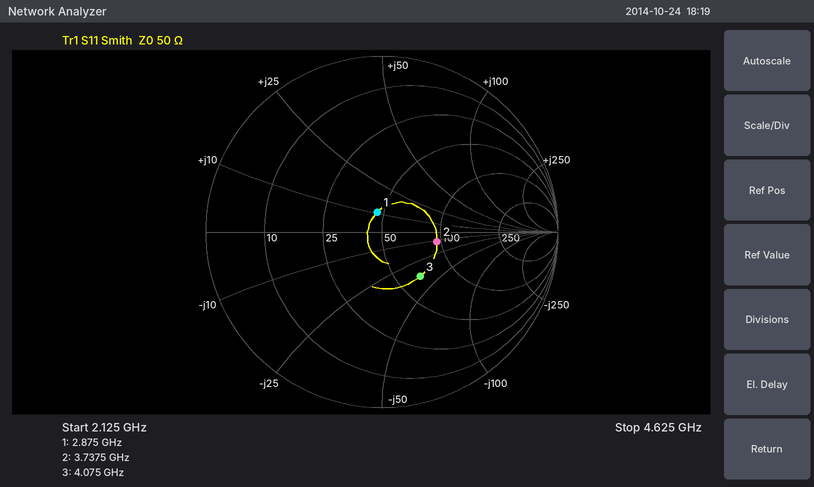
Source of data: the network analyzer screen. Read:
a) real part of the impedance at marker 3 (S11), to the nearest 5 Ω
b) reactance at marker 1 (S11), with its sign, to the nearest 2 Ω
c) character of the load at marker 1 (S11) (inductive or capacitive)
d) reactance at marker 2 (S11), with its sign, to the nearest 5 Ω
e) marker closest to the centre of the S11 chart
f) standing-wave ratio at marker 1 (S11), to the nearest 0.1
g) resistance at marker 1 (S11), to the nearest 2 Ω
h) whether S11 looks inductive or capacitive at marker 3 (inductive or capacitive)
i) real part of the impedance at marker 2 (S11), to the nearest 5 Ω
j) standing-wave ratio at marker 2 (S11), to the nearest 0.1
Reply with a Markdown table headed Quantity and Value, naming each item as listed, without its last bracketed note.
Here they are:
| Quantity | Value |
|---|---|
| real part of the impedance at marker 3 (S11), to the nearest 5 Ω | 65 Ω |
| reactance at marker 1 (S11), with its sign, to the nearest 2 Ω | +10 Ω |
| character of the load at marker 1 (S11) | inductive |
| reactance at marker 2 (S11), with its sign, to the nearest 5 Ω | -10 Ω |
| marker closest to the centre of the S11 chart | marker 1 |
| standing-wave ratio at marker 1 (S11), to the nearest 0.1 | 1.3 |
| resistance at marker 1 (S11), to the nearest 2 Ω | 46 Ω |
| whether S11 looks inductive or capacitive at marker 3 | capacitive |
| real part of the impedance at marker 2 (S11), to the nearest 5 Ω | 95 Ω |
| standing-wave ratio at marker 2 (S11), to the nearest 0.1 | 1.9 |
